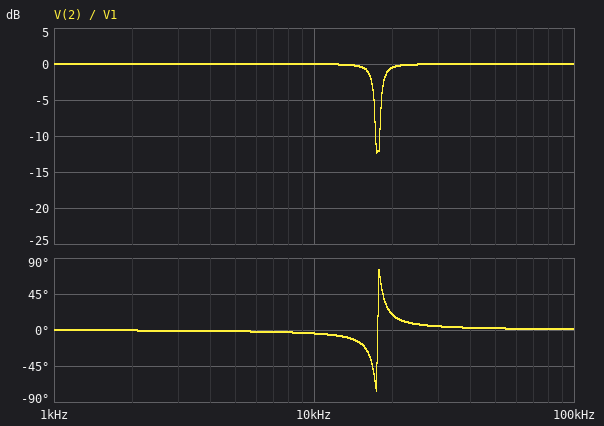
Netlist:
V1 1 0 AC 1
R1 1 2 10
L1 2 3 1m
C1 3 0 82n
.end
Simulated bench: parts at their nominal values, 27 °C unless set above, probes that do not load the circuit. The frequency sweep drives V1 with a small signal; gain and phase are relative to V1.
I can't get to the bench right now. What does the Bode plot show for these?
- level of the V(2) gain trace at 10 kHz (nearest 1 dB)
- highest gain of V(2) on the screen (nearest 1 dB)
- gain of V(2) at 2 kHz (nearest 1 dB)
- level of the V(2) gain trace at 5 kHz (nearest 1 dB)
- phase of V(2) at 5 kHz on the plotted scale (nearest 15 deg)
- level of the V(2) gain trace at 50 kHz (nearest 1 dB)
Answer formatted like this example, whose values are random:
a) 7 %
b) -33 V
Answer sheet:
a) 0 dB
b) 0 dB
c) 0 dB
d) 0 dB
e) 0 deg
f) 0 dB
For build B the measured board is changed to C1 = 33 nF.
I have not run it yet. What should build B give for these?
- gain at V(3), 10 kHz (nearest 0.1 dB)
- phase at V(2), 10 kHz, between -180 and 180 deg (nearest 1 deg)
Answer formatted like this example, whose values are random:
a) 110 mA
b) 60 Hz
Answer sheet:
a) 1.2 dB
b) -1 deg
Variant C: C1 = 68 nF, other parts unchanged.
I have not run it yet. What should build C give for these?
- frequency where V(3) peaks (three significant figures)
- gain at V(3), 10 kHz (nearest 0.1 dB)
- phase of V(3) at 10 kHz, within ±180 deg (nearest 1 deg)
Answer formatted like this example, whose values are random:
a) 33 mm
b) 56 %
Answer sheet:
a) 19.3 kHz
b) 2.7 dB
c) -3 deg
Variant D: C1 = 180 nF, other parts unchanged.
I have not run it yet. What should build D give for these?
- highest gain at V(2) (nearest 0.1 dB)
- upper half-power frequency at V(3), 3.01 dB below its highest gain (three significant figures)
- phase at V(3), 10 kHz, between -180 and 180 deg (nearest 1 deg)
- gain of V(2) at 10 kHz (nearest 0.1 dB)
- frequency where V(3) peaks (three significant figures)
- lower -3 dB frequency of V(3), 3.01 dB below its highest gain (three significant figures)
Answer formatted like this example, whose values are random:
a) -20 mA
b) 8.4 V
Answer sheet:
a) 0 dB
b) 12.6 kHz
c) -21 deg
d) -0.6 dB
e) 11.8 kHz
f) 11.0 kHz
